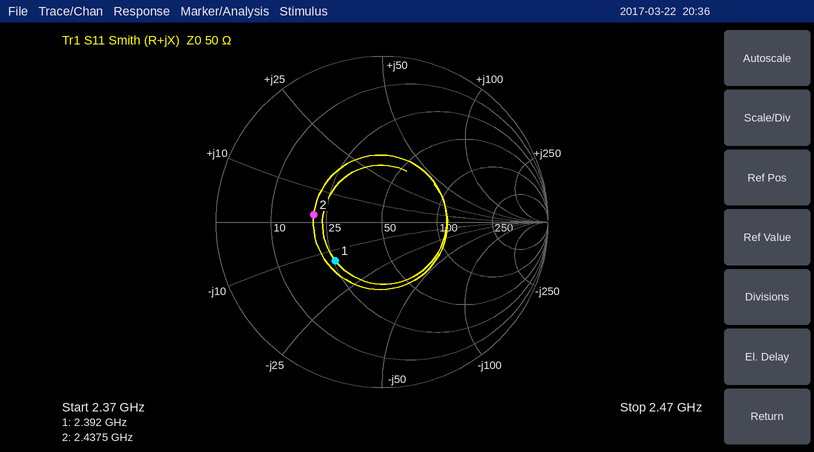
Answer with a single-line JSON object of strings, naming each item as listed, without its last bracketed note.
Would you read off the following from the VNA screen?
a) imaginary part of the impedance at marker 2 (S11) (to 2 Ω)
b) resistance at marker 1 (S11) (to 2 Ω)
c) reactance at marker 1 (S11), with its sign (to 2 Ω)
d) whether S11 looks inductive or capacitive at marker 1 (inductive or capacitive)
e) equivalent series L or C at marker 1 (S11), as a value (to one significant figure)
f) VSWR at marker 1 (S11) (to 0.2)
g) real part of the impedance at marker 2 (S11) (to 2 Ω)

{"imaginary part of the impedance at marker 2 (S11)": "+2 Ω", "resistance at marker 1 (S11)": "26 Ω", "reactance at marker 1 (S11), with its sign": "-14 Ω", "whether S11 looks inductive or capacitive at marker 1": "capacitive", "equivalent series L or C at marker 1 (S11), as a value": "5 pF", "VSWR at marker 1 (S11)": "2.2", "real part of the impedance at marker 2 (S11)": "20 Ω"}
